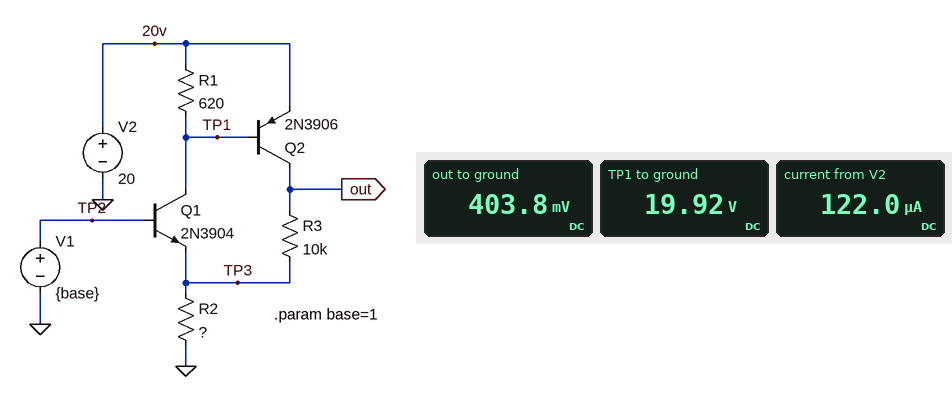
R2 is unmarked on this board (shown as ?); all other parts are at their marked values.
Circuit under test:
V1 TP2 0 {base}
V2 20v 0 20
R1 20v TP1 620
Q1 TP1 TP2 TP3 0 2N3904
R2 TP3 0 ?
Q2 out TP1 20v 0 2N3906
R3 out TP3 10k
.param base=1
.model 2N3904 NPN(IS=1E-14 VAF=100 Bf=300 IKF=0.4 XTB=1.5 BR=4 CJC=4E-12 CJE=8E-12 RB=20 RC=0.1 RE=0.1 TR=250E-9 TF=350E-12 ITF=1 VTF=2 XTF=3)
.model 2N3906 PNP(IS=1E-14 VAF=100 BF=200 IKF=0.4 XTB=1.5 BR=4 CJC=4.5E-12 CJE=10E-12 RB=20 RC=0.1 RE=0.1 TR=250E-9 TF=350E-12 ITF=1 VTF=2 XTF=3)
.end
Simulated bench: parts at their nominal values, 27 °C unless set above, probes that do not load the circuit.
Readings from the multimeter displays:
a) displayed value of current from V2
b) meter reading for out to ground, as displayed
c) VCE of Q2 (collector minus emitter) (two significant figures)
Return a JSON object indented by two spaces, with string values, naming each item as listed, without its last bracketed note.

{
  "displayed value of current from V2": "122.0 µA",
  "meter reading for out to ground, as displayed": "403.8 mV",
  "VCE of Q2 (collector minus emitter)": "-20 V"
}
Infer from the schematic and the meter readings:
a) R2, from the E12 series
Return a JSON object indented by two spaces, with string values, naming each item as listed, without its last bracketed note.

{
  "R2, from the E12 series": "3.3 kΩ"
}
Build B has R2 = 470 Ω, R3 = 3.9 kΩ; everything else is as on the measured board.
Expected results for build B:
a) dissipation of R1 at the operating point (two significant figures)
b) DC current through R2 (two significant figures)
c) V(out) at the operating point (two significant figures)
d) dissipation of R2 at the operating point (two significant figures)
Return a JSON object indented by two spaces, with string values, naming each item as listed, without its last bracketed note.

{
  "dissipation of R1 at the operating point": "350 µW",
  "DC current through R2": "760 µA",
  "V(out) at the operating point": "360 mV",
  "dissipation of R2 at the operating point": "270 µW"
}
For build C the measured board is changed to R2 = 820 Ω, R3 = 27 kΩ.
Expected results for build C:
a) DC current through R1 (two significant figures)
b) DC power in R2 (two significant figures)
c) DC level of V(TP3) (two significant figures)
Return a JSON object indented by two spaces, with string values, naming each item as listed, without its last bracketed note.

{
  "DC current through R1": "450 µA",
  "DC power in R2": "170 µW",
  "DC level of V(TP3)": "370 mV"
}
